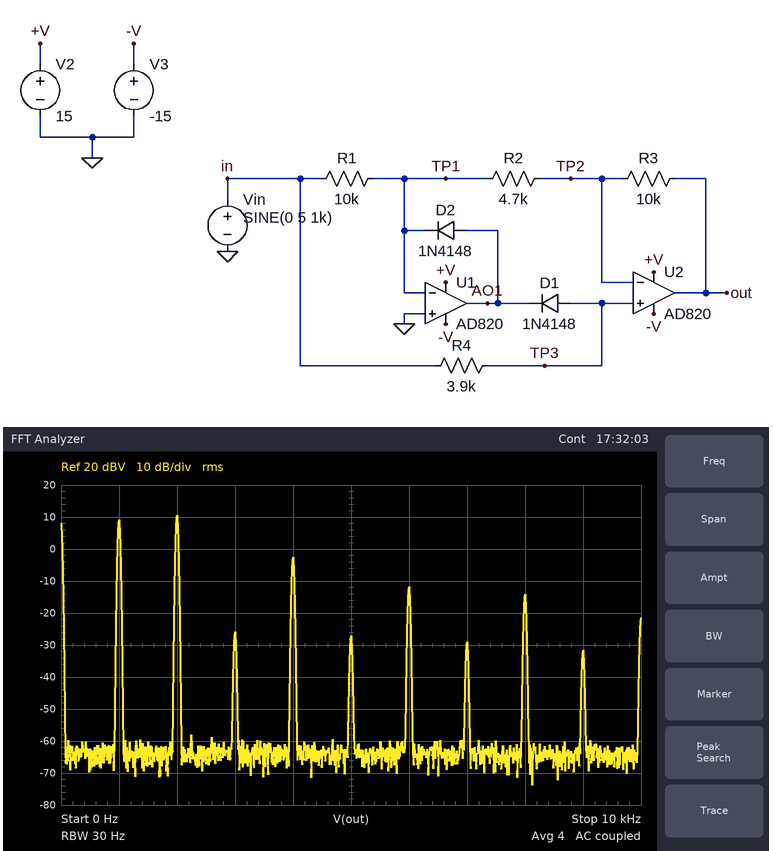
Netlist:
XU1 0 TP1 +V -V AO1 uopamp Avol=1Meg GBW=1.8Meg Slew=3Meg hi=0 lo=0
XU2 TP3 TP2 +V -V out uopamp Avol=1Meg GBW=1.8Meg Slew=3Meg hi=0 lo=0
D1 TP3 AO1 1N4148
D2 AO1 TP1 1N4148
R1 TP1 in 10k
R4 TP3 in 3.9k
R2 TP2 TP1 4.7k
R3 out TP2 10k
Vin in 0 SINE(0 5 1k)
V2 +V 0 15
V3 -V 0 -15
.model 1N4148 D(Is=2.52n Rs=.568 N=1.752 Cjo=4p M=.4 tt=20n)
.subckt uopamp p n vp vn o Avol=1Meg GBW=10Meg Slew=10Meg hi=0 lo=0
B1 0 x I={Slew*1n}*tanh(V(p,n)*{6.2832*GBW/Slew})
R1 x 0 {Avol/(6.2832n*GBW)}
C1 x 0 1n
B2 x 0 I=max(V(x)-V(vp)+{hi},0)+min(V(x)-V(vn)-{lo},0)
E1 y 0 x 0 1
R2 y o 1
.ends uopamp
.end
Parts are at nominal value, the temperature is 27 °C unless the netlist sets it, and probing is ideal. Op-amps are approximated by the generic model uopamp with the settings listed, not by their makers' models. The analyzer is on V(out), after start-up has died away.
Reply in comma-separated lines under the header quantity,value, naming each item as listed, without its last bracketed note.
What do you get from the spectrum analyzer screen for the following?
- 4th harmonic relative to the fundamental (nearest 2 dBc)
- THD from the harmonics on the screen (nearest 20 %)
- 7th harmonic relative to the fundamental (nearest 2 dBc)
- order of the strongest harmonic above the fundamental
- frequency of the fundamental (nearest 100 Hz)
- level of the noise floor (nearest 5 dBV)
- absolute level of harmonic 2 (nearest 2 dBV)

quantity,value
4th harmonic relative to the fundamental,-12 dBc
THD from the harmonics on the screen,120 %
7th harmonic relative to the fundamental,-38 dBc
order of the strongest harmonic above the fundamental,2
frequency of the fundamental,1.0 kHz
level of the noise floor,-65 dBV
absolute level of harmonic 2,10 dBV
